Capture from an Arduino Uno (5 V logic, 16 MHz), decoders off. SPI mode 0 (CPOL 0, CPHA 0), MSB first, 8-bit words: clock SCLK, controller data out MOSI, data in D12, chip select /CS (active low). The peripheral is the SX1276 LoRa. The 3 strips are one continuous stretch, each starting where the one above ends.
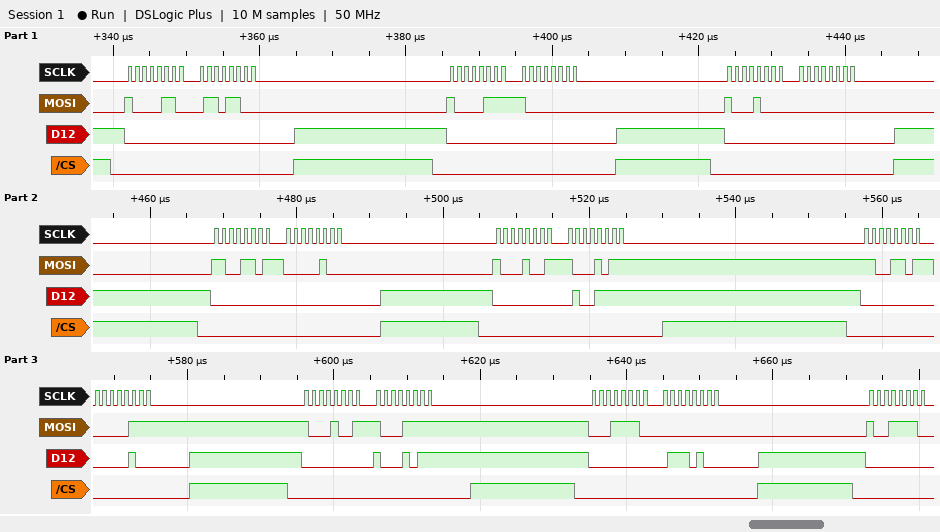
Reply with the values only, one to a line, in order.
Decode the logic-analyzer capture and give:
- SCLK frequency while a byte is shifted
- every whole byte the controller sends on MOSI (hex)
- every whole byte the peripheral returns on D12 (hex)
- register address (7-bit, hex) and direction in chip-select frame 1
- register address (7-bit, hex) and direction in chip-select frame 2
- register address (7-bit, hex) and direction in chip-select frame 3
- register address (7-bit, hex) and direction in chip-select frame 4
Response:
1 MHz
0x86 0x6C 0x87 0x80 0x88 0x00 0xCD 0x04 0x89 0x8B 0xCD 0x07 0x89 0x8F 0x1E 0x00 0x9E
0x00 0x00 0x00 0x00 0x00 0x00 0x00 0x00 0x00 0x4F 0x00 0x04 0x00 0x8B 0x00 0x74 0x00
0x06 write
0x07 write
0x08 write
0x4D write
